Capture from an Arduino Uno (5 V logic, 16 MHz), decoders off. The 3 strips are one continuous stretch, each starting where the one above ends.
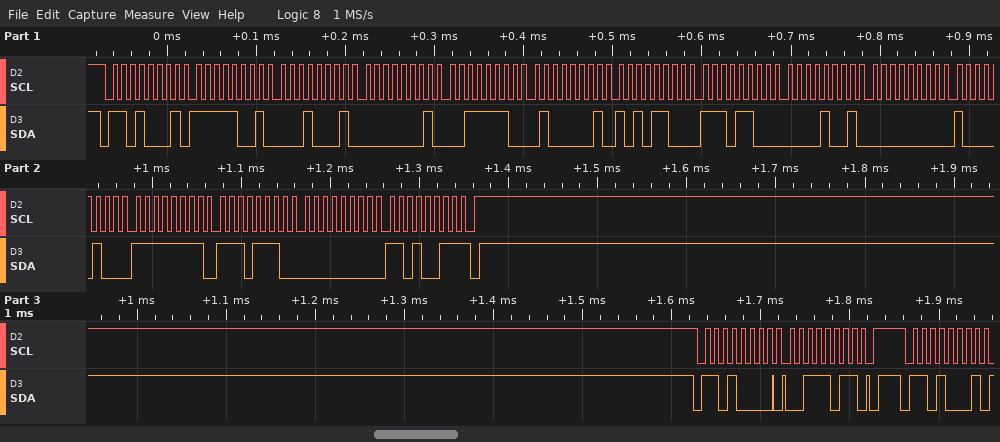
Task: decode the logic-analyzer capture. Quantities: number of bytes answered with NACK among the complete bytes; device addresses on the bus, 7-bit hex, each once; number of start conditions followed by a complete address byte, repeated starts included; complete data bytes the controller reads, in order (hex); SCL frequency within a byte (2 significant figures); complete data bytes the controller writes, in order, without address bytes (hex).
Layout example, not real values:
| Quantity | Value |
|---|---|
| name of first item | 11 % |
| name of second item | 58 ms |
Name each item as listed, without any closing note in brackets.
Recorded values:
| Quantity | Value |
|---|---|
| number of bytes answered with NACK among the complete bytes | 1 |
| device addresses on the bus, 7-bit hex, each once | 0x68 |
| number of start conditions followed by a complete address byte, repeated starts included | 3 |
| complete data bytes the controller reads, in order | F9 11 01 3E 41 AC EC 09 00 84 FF EE 00 D3 |
| SCL frequency within a byte | 100 kHz |
| complete data bytes the controller writes, in order, without address bytes | 3B |
